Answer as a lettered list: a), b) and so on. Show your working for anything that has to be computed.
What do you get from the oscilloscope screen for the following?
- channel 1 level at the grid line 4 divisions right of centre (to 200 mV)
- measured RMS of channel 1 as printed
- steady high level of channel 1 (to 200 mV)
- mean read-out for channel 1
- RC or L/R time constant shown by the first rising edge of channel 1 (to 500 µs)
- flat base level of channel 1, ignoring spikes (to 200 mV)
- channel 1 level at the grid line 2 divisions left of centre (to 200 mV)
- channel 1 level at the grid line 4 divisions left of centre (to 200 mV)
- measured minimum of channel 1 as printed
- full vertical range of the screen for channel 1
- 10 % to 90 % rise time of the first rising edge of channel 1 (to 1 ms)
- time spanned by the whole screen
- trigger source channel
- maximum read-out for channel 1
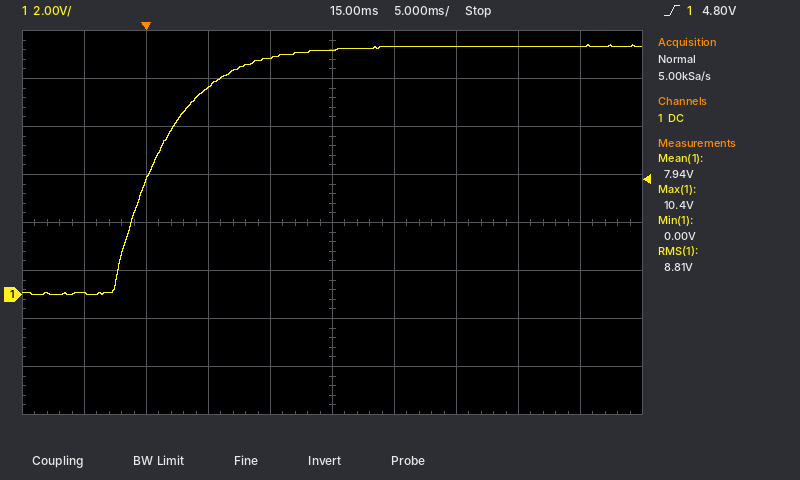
a) 10.4 V
b) 8.81 V
c) 10.4 V
d) 7.94 V
e) 9 ms / 2.2 ≈ 4.09 ms, so 4.0 ms to the nearest 500 µs
f) 0.0 V
g) 8.6 V
h) 0.0 V
i) 0.00 V
j) 16 V
k) 9 ms
l) 50 ms
m) channel 1
n) 10.4 V
